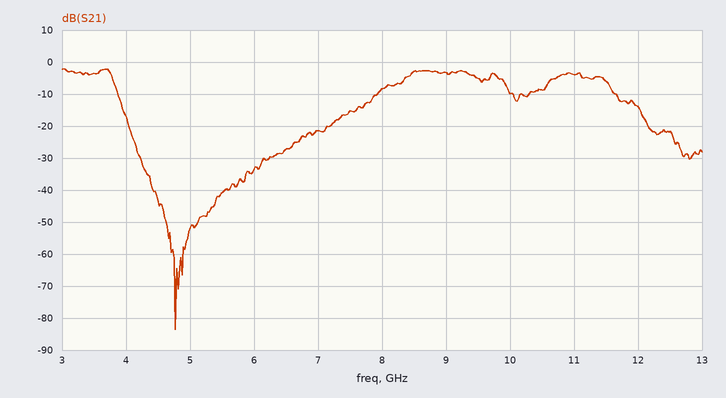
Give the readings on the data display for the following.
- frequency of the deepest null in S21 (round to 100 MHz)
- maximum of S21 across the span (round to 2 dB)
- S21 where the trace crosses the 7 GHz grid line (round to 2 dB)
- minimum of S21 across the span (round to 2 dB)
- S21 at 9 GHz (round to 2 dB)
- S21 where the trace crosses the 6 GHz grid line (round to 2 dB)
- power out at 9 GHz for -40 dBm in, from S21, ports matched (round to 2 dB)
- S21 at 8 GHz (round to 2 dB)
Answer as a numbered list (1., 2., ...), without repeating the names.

1. 4.8 GHz
2. -2 dB
3. -22 dB
4. -84 dB
5. -4 dB
6. -34 dB
7. -44 dBm
8. -8 dB
